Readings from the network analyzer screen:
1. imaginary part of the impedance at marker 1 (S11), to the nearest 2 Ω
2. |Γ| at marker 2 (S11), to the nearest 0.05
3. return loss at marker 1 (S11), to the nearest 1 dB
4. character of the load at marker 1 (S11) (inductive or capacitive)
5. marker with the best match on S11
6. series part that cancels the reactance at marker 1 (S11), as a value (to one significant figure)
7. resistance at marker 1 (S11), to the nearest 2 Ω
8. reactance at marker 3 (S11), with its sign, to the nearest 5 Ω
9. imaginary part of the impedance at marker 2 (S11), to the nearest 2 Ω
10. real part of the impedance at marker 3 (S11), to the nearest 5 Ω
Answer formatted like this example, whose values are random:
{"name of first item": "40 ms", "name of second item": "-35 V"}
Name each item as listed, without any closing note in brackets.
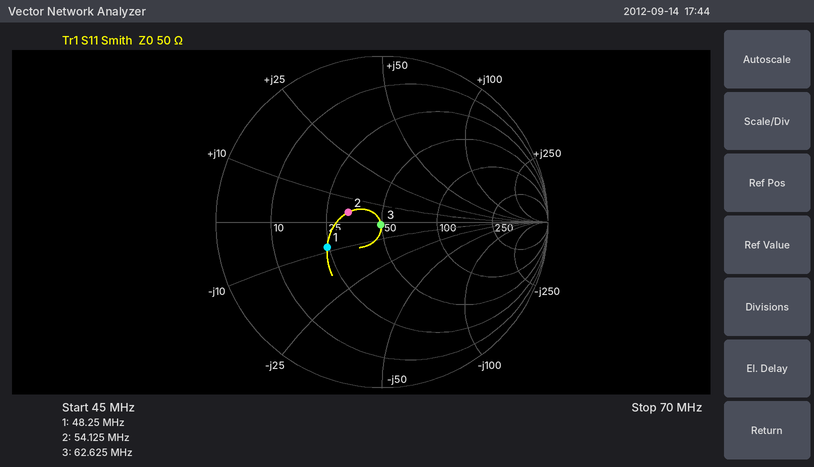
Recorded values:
{"imaginary part of the impedance at marker 1 (S11), to the nearest 2 Ω": "-8 Ω", "|Γ| at marker 2 (S11), to the nearest 0.05": "0.20", "return loss at marker 1 (S11), to the nearest 1 dB": "9 dB", "character of the load at marker 1 (S11)": "capacitive", "marker with the best match on S11": "marker 3", "series part that cancels the reactance at marker 1 (S11), as a value": "30 nH", "resistance at marker 1 (S11), to the nearest 2 Ω": "24 Ω", "reactance at marker 3 (S11), with its sign, to the nearest 5 Ω": "0 Ω", "imaginary part of the impedance at marker 2 (S11), to the nearest 2 Ω": "+4 Ω", "real part of the impedance at marker 3 (S11), to the nearest 5 Ω": "50 Ω"}
